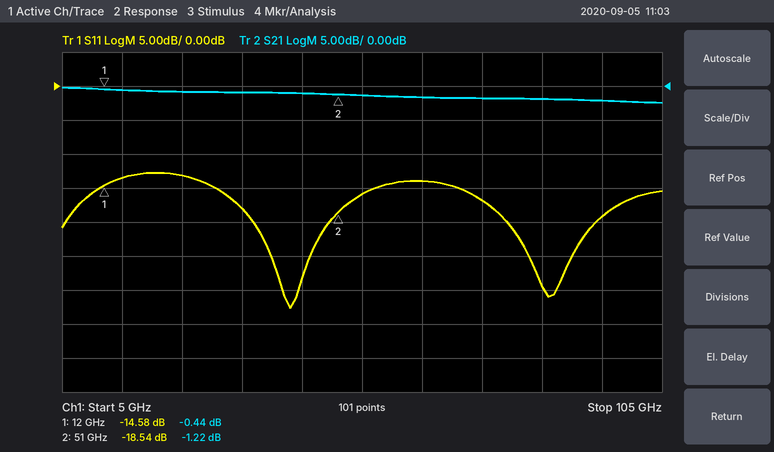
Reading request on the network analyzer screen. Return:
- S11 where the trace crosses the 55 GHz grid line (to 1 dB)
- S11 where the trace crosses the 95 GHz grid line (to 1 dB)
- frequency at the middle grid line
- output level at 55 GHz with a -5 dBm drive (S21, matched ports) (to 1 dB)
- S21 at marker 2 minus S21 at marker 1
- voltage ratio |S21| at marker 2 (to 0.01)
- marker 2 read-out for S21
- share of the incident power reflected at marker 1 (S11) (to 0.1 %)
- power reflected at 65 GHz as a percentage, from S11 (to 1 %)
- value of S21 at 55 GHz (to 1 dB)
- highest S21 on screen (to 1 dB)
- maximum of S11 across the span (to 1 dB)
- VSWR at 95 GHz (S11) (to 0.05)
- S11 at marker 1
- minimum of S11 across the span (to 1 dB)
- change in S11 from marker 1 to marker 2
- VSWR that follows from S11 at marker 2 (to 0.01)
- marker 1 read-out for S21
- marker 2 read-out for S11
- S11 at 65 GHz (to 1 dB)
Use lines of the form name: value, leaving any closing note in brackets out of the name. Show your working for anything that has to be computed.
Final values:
S11 where the trace crosses the 55 GHz grid line: -16 dB
S11 where the trace crosses the 95 GHz grid line: -19 dB
frequency at the middle grid line: 55 GHz
output level at 55 GHz with a -5 dBm drive (S21, matched ports): -5 dBm + (-1 dB) = -6 dBm
S21 at marker 2 minus S21 at marker 1: -1.22 − (-0.44) = -0.78 dB
voltage ratio |S21| at marker 2: 10^(-1.22/20) ≈ 0.87
marker 2 read-out for S21: -1.22 dB
share of the incident power reflected at marker 1 (S11): 10^(-14.58/10) ≈ 3.5 %
power reflected at 65 GHz as a percentage, from S11: 10^(-14/10) ≈ 4 %
value of S21 at 55 GHz: -1 dB
highest S21 on screen: 0 dB
maximum of S11 across the span: -13 dB
VSWR at 95 GHz (S11): |Γ| = 10^(-19/20) = 0.1122; VSWR = (1 + 0.1122)/(1 − 0.1122) ≈ 1.25
S11 at marker 1: -14.58 dB
minimum of S11 across the span: -33 dB
change in S11 from marker 1 to marker 2: -18.54 − (-14.58) = -3.96 dB
VSWR that follows from S11 at marker 2: (1 + 0.1183)/(1 − 0.1183) ≈ 1.27
marker 1 read-out for S21: -0.44 dB
marker 2 read-out for S11: -18.54 dB
S11 at 65 GHz: -14 dB
